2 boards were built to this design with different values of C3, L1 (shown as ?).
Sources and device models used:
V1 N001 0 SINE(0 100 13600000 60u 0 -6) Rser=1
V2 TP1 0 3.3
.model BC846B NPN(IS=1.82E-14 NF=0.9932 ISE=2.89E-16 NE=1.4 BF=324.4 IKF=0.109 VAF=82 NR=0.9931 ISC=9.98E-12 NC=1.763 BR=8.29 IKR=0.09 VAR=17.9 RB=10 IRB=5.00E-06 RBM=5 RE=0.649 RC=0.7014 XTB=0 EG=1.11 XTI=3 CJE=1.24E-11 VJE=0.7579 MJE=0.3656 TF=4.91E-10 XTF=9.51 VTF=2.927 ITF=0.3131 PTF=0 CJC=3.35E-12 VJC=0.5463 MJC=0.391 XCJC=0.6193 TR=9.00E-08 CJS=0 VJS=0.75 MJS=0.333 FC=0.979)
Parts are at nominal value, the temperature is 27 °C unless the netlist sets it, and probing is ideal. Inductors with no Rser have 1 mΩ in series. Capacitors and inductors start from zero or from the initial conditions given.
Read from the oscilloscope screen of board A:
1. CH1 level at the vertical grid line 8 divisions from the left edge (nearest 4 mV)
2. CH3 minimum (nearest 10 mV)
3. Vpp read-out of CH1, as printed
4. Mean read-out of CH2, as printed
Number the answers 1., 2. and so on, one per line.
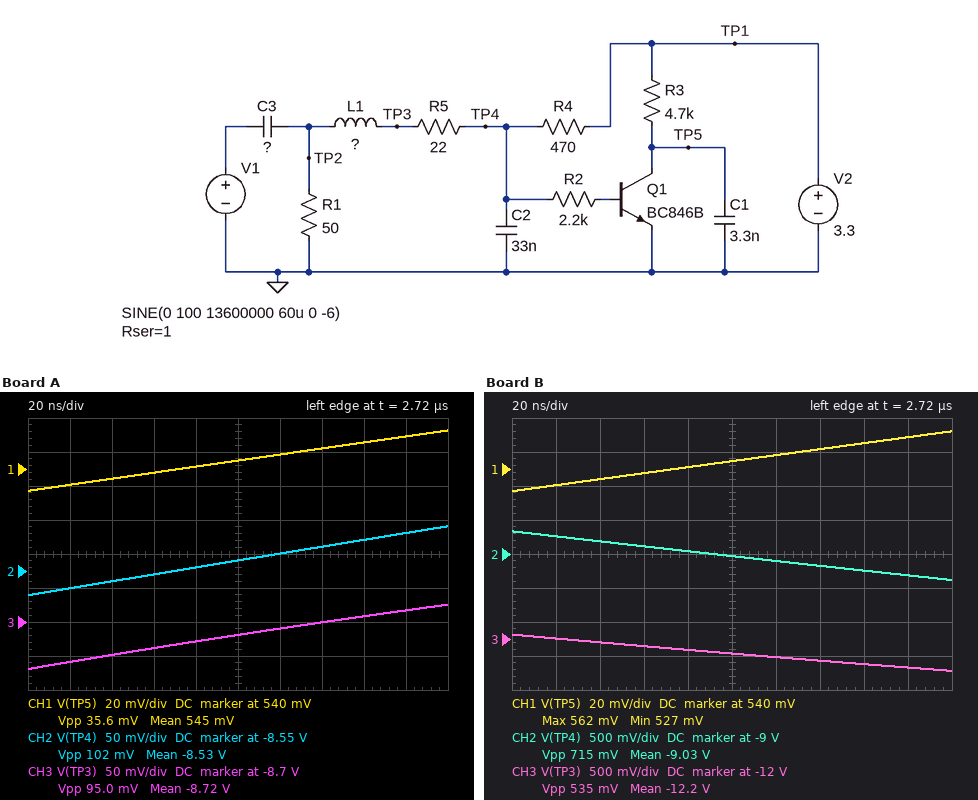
1. 556 mV
2. -8.77 V
3. 35.6 mV
4. -8.53 V
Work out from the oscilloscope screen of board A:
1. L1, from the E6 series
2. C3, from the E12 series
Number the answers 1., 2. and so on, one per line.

1. 6.8 µH
2. 560 nF
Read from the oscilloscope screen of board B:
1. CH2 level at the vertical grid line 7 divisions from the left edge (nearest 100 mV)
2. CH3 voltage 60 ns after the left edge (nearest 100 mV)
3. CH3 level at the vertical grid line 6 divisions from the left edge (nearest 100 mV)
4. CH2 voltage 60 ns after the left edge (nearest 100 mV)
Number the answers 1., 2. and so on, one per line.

1. -9.2 V
2. -12.1 V
3. -12.3 V
4. -8.9 V
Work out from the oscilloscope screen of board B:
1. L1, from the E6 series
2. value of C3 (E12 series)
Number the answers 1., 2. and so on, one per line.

1. 68 µH
2. 1.2 µF
